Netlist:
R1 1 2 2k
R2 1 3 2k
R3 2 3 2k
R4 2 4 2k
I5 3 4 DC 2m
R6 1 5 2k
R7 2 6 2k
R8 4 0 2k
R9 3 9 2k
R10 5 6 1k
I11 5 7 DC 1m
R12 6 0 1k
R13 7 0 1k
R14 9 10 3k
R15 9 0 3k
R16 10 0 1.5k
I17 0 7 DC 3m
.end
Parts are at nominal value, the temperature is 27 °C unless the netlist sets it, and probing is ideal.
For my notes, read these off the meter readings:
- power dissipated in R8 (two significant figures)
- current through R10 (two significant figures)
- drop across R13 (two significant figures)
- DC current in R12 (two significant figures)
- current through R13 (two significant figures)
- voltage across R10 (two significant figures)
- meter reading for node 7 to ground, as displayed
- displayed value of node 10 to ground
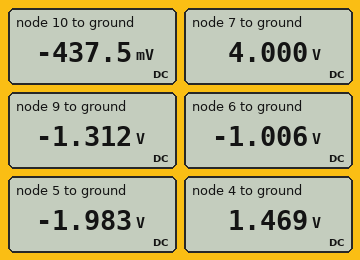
1.1 mW
980 µA
4.0 V
1.0 mA
4.0 mA
980 mV
4.000 V
-437.5 mV
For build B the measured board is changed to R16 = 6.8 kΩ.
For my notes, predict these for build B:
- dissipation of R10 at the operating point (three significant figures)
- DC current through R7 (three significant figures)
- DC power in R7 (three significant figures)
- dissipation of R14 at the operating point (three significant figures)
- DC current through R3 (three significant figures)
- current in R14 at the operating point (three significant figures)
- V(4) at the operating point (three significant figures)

989 µW
46.5 µA
4.32 µW
75.2 µW
885 µA
158 µA
1.43 V
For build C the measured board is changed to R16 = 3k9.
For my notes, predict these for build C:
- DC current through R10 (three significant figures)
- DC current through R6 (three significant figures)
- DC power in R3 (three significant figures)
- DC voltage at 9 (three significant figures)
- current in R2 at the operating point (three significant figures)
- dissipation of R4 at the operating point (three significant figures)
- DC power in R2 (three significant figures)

988 µA
12.2 µA
1.52 mW
-1.46 V
430 µA
3.26 mW
370 µW
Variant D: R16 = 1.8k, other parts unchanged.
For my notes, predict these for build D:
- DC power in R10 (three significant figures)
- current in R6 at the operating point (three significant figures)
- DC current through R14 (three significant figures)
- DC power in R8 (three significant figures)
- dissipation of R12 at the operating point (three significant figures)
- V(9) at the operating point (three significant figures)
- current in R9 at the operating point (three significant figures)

959 µW
20.7 µA
278 µA
1.07 mW
1.02 mW
-1.34 V
724 µA
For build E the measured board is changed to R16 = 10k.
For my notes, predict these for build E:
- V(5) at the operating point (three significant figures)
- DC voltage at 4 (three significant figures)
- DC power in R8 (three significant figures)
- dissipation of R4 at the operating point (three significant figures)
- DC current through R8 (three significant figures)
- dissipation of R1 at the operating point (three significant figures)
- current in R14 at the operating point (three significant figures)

-2.05 V
1.42 V
1.01 mW
3.32 mW
712 µA
399 µW
124 µA
